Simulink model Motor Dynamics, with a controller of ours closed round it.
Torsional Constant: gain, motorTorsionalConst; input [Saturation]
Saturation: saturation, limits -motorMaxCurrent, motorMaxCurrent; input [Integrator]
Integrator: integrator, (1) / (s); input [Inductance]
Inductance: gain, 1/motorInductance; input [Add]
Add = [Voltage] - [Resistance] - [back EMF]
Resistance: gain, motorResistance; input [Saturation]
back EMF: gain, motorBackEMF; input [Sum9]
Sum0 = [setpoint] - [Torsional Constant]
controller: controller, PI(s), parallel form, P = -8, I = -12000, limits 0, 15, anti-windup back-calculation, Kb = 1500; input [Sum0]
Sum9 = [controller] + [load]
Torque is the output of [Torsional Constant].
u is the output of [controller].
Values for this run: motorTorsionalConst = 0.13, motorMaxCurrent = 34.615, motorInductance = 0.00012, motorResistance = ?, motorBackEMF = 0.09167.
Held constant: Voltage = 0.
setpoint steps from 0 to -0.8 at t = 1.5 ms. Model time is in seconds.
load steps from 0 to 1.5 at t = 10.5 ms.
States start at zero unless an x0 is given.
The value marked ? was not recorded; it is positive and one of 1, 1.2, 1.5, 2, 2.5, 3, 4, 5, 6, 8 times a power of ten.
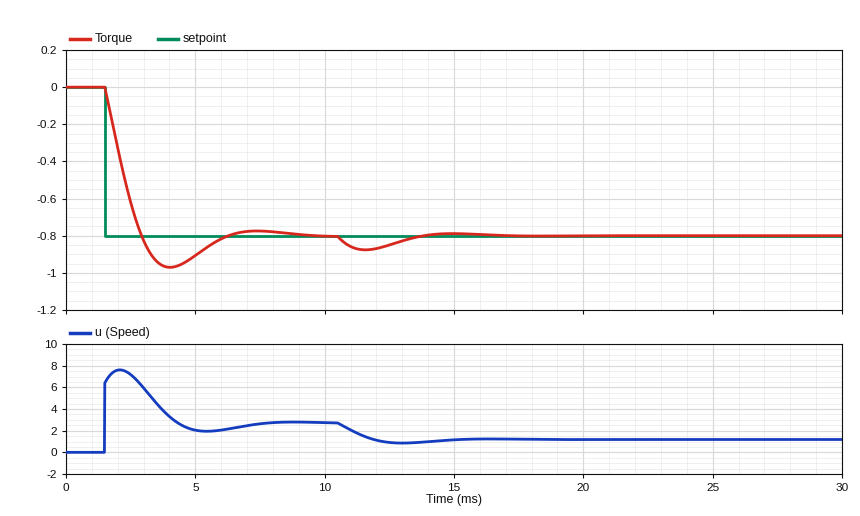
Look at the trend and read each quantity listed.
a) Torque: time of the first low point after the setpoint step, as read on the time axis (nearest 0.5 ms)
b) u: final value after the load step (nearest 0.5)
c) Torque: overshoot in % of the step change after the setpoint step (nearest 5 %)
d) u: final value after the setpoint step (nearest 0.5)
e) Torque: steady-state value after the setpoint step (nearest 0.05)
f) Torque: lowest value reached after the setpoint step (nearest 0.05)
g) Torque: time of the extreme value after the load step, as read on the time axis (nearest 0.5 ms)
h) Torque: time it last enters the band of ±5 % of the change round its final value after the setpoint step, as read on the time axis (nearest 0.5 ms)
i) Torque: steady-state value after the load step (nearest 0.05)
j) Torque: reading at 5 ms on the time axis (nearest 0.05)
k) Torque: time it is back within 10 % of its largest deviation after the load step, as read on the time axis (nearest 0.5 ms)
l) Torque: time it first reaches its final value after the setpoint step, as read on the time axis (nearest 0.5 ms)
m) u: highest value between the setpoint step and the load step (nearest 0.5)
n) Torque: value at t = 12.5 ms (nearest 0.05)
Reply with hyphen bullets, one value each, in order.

- 4.0 ms
- 1.0
- 20 %
- 2.5
- -0.80
- -0.95
- 11.5 ms
- 5.5 ms
- -0.80
- -0.90
- 16.0 ms
- 3.0 ms
- 7.5
- -0.85
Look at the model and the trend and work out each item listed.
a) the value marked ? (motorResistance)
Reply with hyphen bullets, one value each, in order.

- 0.04
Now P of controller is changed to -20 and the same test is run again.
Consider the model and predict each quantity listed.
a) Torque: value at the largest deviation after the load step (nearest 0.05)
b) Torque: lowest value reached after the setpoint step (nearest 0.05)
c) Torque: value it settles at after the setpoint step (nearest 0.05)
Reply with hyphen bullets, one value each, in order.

- -0.85
- -0.85
- -0.80
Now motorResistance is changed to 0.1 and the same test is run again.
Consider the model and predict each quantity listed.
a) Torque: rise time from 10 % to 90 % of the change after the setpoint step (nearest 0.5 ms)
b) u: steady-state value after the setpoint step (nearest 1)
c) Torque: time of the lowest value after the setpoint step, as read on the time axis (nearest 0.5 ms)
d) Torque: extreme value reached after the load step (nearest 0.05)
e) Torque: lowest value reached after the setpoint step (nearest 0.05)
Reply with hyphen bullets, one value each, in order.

- 1.5 ms
- 7
- 4.5 ms
- -0.85
- -0.85
